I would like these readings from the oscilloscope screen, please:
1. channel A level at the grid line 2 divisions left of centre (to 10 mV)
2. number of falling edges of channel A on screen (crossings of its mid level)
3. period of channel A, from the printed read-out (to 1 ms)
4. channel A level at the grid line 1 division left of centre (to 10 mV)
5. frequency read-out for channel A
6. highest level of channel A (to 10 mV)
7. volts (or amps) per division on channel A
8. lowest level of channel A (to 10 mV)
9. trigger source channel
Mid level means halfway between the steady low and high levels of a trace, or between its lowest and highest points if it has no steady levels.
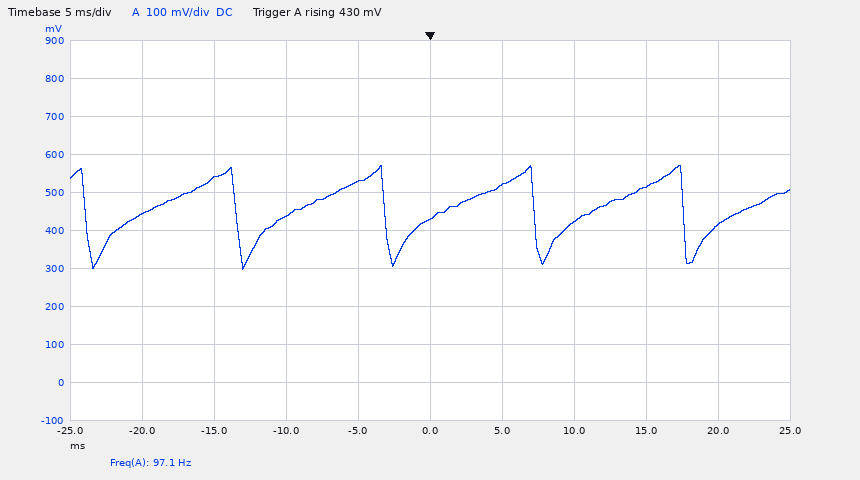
440 mV
5
10 ms
530 mV
97.1 Hz
570 mV
100 mV
300 mV
channel A
